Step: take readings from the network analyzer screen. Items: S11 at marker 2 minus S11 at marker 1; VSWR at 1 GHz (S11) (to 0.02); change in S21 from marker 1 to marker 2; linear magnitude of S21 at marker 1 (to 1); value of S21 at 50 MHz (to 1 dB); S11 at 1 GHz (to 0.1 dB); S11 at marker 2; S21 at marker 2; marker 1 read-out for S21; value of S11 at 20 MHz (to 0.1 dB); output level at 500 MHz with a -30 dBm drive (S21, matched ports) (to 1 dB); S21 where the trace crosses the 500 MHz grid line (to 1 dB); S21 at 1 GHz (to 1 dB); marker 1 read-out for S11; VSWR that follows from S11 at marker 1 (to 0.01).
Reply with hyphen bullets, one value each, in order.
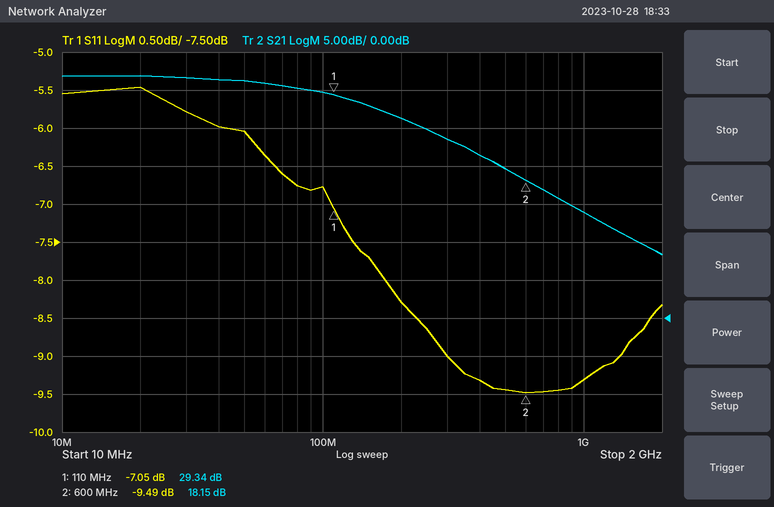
- -2.44 dB
- 2.04
- -11.19 dB
- 29
- 31 dB
- -9.3 dB
- -9.49 dB
- 18.15 dB
- 29.34 dB
- -5.5 dB
- -10 dBm
- 20 dB
- 14 dB
- -7.05 dB
- 2.60
